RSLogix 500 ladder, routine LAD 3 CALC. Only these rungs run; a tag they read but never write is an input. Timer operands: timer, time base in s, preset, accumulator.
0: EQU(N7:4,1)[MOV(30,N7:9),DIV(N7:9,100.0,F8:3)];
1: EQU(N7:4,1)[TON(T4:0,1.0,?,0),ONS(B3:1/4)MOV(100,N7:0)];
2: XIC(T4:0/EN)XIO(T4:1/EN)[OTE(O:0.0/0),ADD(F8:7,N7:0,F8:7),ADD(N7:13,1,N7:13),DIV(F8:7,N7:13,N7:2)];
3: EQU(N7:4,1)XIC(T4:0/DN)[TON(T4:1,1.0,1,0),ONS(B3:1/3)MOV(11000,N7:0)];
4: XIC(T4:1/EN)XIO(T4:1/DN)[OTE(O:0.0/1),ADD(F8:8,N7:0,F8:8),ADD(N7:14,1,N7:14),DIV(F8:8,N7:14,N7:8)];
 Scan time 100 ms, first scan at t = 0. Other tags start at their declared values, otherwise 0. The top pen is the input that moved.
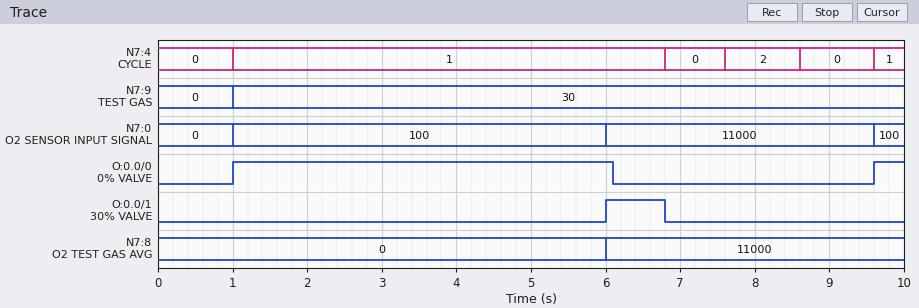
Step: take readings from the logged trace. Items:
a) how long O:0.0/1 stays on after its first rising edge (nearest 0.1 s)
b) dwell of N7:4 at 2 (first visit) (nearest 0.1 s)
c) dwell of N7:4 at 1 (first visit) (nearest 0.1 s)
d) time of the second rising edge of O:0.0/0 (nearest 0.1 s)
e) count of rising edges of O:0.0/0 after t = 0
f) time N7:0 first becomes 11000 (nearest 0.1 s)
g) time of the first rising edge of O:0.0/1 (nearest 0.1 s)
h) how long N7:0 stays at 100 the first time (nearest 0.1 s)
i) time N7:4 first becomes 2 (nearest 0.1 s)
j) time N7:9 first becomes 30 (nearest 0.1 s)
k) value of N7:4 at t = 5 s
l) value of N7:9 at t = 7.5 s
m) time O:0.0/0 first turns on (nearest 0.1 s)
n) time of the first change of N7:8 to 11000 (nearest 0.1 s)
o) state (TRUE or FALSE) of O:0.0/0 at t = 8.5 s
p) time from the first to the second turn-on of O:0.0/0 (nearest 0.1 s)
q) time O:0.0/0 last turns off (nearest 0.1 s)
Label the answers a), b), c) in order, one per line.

a) 0.8 s
b) 1.0 s
c) 5.8 s
d) 9.6 s
e) 2
f) 6.0 s
g) 6.0 s
h) 5.0 s
i) 7.6 s
j) 1.0 s
k) 1
l) 30
m) 1.0 s
n) 6.0 s
o) FALSE
p) 8.6 s
q) 6.1 s
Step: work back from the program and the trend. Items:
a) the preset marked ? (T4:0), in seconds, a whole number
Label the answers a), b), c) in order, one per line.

a) 5 s
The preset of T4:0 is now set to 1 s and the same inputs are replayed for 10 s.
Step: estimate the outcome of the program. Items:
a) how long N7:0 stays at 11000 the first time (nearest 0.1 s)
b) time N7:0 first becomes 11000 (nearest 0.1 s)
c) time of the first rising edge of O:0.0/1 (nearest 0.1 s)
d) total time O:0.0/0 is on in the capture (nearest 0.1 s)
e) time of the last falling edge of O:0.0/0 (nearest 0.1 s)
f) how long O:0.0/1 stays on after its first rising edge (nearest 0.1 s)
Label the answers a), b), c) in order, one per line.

a) 7.6 s
b) 2.0 s
c) 2.0 s
d) 1.5 s
e) 2.1 s
f) 1.0 s
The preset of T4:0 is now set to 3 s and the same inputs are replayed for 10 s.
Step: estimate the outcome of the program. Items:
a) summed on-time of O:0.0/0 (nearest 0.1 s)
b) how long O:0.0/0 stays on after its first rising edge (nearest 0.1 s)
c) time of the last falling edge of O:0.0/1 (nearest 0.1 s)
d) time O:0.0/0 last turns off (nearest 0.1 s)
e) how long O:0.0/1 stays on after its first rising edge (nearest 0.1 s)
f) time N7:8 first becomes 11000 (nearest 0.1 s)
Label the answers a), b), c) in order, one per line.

a) 3.5 s
b) 3.1 s
c) 5.0 s
d) 4.1 s
e) 1.0 s
f) 4.0 s
